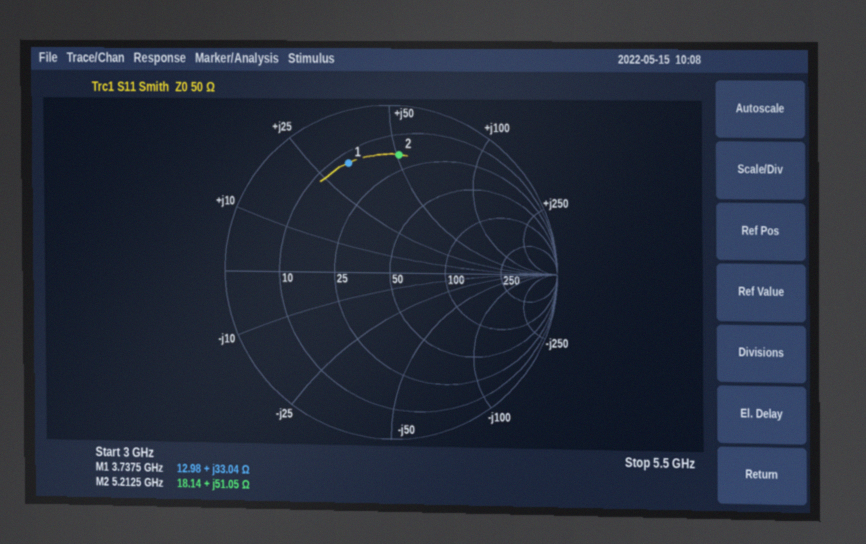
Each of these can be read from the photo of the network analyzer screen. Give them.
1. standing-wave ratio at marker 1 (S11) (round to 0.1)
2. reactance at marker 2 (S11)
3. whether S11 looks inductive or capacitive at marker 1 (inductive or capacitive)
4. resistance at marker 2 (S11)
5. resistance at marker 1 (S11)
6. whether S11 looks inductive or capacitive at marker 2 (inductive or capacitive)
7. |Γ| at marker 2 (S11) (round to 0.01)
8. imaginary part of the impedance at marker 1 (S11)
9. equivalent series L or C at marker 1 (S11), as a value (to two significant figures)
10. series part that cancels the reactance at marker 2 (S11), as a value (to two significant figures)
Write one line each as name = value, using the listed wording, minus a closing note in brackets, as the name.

standing-wave ratio at marker 1 (S11) = 5.6
reactance at marker 2 = +51.05 Ω
whether S11 looks inductive or capacitive at marker 1 = inductive
resistance at marker 2 = 18.14 Ω
resistance at marker 1 = 12.98 Ω
whether S11 looks inductive or capacitive at marker 2 = inductive
|Γ| at marker 2 (S11) = 0.71
imaginary part of the impedance at marker 1 = +33.04 Ω
equivalent series L or C at marker 1 (S11), as a value = 1.4 nH
series part that cancels the reactance at marker 2 (S11), as a value = 600 fF
